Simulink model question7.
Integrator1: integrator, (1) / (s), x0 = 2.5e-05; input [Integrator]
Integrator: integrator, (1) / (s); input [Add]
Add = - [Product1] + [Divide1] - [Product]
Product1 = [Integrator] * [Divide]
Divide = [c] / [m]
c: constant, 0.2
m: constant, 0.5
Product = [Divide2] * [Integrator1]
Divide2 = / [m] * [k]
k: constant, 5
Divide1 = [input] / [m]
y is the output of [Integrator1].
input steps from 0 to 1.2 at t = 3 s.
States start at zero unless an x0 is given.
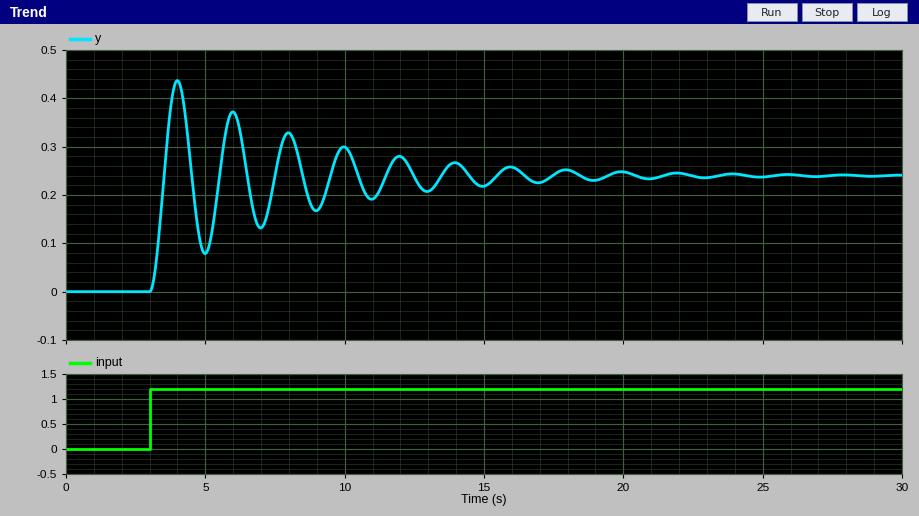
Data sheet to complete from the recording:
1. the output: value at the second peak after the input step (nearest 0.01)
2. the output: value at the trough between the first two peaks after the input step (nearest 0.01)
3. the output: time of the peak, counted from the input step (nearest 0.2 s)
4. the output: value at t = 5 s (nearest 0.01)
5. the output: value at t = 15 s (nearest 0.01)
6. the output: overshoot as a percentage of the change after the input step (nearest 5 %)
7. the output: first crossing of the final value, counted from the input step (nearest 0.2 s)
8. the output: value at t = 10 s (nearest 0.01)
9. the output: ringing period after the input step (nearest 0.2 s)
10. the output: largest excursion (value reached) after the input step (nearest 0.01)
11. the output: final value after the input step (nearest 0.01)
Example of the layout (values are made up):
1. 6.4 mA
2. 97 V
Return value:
1. 0.37
2. 0.08
3. 1.0 s
4. 0.08
5. 0.22
6. 80 %
7. 0.6 s
8. 0.30
9. 2.0 s
10. 0.44
11. 0.24
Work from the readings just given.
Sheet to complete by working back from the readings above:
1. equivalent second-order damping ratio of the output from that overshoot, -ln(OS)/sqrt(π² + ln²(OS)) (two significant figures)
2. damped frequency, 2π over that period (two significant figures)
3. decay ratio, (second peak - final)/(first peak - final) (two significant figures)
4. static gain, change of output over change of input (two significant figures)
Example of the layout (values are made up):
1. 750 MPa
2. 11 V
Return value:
1. 0.071
2. 3.1 rad/s
3. 0.65
4. 0.20
